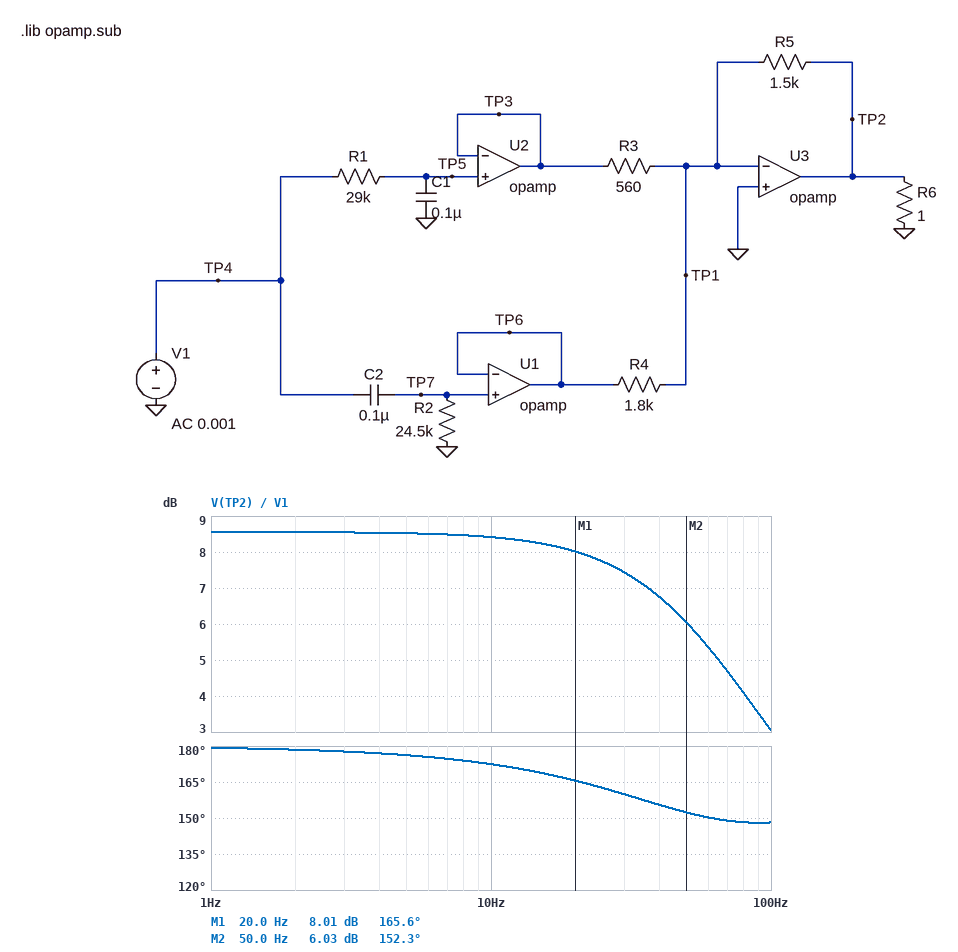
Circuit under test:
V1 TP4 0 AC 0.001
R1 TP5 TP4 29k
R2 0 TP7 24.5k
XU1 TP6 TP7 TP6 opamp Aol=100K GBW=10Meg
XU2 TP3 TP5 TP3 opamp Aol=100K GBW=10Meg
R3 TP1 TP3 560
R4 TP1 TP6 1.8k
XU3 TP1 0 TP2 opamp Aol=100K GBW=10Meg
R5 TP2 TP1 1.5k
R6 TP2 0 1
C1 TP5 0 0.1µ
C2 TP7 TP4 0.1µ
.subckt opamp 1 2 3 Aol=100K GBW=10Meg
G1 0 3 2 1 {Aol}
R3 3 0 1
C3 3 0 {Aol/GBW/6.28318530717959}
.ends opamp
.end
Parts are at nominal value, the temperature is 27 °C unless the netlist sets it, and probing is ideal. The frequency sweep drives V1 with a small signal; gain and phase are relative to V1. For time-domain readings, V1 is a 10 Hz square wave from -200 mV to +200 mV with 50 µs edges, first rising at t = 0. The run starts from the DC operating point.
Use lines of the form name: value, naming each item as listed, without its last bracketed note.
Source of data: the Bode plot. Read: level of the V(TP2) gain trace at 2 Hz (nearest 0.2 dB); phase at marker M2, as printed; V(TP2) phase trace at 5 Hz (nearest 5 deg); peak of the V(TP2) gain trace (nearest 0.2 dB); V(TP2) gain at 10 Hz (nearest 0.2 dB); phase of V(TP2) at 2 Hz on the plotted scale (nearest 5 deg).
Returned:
level of the V(TP2) gain trace at 2 Hz: 8.6 dB
phase at marker M2, as printed: 152.3 deg
V(TP2) phase trace at 5 Hz: 175 deg
peak of the V(TP2) gain trace: 8.6 dB
V(TP2) gain at 10 Hz: 8.4 dB
phase of V(TP2) at 2 Hz on the plotted scale: 180 deg
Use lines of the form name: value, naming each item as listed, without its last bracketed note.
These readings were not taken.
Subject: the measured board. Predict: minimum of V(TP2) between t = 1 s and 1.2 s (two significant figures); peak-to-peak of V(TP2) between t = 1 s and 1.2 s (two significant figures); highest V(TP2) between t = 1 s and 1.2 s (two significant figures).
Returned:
minimum of V(TP2) between t = 1 s and 1.2 s: -540 mV
peak-to-peak of V(TP2) between t = 1 s and 1.2 s: 1.1 V
highest V(TP2) between t = 1 s and 1.2 s: 540 mV
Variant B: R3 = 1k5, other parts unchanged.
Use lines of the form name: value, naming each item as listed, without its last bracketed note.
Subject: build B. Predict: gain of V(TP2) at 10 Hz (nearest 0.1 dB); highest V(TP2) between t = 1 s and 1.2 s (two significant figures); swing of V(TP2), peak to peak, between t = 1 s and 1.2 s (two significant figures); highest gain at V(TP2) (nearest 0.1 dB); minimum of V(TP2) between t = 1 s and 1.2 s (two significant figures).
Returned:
gain of V(TP2) at 10 Hz: -0.1 dB
highest V(TP2) between t = 1 s and 1.2 s: 200 mV
swing of V(TP2), peak to peak, between t = 1 s and 1.2 s: 400 mV
highest gain at V(TP2): 0 dB
minimum of V(TP2) between t = 1 s and 1.2 s: -200 mV
